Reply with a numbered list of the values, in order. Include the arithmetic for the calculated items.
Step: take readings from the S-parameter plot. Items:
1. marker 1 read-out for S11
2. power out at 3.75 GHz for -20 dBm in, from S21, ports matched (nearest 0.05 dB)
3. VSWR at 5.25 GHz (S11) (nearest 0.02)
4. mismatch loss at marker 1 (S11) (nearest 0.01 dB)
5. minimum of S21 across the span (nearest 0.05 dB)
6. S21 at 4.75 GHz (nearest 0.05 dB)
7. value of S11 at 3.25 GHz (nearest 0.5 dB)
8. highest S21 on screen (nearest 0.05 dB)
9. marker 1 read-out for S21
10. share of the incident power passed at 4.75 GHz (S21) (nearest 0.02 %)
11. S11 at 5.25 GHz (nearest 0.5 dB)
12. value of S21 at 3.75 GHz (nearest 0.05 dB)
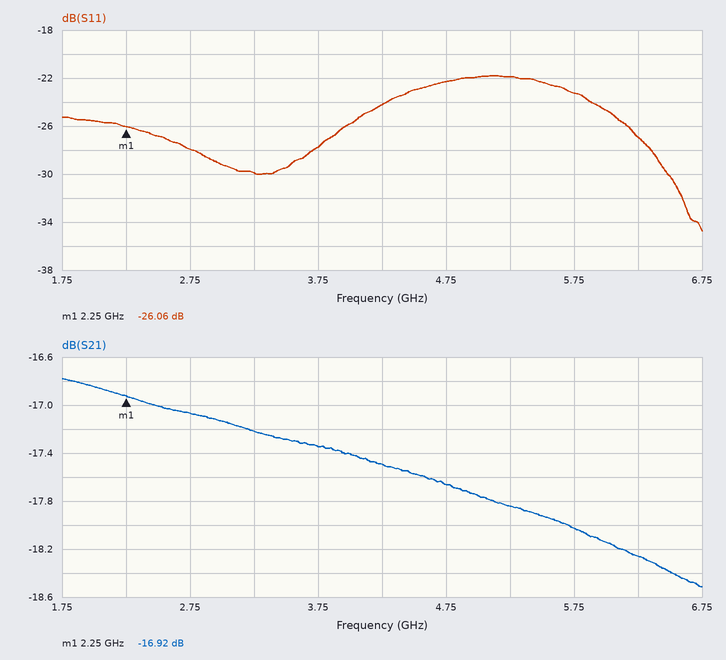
1. -26.06 dB
2. -20 dBm + (-17.35 dB) = -37.35 dBm
3. |Γ| = 10^(-22/20) = 0.0794; VSWR = (1 + 0.0794)/(1 − 0.0794) ≈ 1.17, so 1.18 to the nearest 0.02
4. −10 log10(1 − 10^(-26.06/10)) ≈ 0.01 dB
5. -18.50 dB
6. -17.65 dB
7. -30.0 dB
8. -16.80 dB
9. -16.92 dB
10. 10^(-17.65/10) ≈ 1.72 %
11. -22.0 dB
12. -17.35 dB
